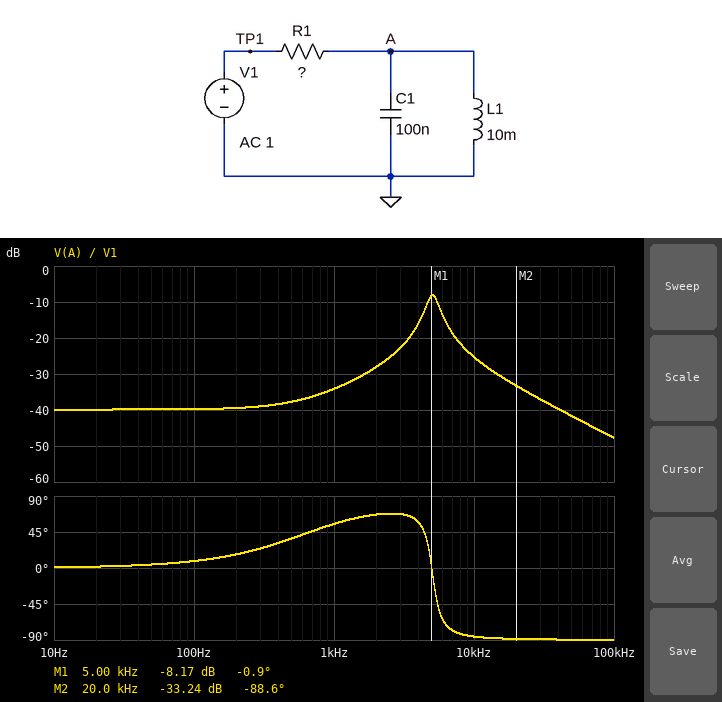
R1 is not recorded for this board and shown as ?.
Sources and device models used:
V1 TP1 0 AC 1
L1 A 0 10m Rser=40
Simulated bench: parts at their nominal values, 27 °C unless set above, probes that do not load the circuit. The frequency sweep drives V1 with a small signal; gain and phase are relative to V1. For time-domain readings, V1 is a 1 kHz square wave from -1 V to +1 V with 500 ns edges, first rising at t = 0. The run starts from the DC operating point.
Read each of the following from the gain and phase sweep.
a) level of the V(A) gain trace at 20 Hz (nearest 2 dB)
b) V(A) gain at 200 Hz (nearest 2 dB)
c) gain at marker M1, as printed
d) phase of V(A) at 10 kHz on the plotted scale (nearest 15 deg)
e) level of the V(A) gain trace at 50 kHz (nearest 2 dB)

-40 dB
-40 dB
-8.17 dB
-90 deg
-42 dB
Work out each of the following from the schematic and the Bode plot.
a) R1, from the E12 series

3.9 kΩ
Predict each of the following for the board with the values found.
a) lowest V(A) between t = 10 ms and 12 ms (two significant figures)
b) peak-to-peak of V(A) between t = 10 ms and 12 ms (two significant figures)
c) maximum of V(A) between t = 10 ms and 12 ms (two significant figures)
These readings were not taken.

-180 mV
360 mV
180 mV
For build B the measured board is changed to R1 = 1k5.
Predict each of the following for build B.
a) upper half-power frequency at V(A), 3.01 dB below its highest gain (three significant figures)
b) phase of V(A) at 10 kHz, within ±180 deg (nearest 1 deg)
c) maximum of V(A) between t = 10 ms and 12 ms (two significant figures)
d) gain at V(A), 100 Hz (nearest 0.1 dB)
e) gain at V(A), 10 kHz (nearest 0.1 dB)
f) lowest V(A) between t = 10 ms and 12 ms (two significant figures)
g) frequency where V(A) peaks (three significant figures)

6.01 kHz
-81 deg
370 mV
-31.6 dB
-17.1 dB
-370 mV
5.10 kHz
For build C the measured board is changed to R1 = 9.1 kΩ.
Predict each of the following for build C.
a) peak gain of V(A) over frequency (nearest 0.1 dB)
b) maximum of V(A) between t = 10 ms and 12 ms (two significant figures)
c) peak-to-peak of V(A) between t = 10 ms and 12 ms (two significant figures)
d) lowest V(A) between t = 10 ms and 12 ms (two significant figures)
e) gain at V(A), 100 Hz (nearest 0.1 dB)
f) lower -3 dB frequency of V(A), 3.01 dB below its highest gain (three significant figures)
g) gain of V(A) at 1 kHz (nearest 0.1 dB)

-13.3 dB
89 mV
180 mV
-89 mV
-47.1 dB
4.65 kHz
-41.4 dB
